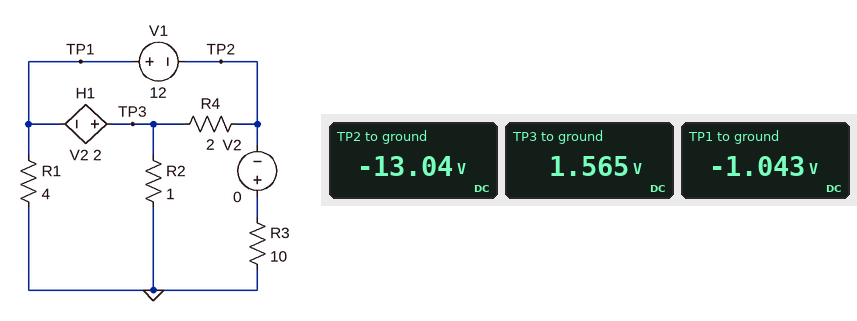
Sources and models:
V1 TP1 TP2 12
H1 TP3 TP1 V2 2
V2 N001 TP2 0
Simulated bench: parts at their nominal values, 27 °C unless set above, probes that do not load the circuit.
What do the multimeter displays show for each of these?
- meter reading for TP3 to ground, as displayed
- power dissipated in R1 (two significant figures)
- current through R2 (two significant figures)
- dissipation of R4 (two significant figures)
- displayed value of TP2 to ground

1.565 V
270 mW
1.6 A
110 W
-13.04 V
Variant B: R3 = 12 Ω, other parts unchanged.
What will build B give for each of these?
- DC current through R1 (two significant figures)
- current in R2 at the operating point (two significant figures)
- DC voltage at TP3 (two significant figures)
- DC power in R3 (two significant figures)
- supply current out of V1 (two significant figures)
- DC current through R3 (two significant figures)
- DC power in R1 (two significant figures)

210 mA
1.3 A
1.3 V
14 W
8.1 A
1.1 A
180 mW
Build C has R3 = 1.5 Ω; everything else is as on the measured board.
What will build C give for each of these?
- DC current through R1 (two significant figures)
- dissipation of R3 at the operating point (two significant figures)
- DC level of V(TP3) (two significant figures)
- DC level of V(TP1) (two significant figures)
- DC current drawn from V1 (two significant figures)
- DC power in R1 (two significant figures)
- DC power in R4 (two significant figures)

3.4 A
440 W
21 V
-14 V
40 A
47 W
1.1 kW
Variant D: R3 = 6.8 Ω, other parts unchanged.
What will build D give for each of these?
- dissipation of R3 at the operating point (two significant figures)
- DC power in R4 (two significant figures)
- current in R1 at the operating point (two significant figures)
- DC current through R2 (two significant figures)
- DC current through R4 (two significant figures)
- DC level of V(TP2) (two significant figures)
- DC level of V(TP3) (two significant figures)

27 W
130 W
400 mA
2.4 A
8.0 A
-14 V
2.4 V
